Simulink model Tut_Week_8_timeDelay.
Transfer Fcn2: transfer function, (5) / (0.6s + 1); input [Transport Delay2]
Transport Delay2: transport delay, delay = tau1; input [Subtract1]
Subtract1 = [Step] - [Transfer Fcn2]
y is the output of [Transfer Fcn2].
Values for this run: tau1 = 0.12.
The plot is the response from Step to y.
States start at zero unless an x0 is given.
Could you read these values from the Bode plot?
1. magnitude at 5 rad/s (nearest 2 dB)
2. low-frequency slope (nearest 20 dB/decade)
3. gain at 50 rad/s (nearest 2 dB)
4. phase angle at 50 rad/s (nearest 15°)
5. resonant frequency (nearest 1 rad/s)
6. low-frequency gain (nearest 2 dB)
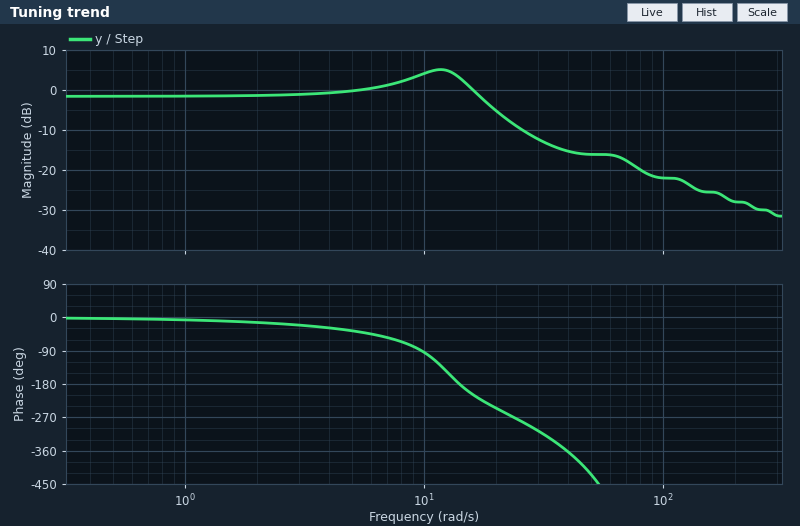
0 dB
0 dB/decade
-16 dB
-420°
12 rad/s
-2 dB
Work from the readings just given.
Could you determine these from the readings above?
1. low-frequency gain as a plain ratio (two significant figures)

0.79
